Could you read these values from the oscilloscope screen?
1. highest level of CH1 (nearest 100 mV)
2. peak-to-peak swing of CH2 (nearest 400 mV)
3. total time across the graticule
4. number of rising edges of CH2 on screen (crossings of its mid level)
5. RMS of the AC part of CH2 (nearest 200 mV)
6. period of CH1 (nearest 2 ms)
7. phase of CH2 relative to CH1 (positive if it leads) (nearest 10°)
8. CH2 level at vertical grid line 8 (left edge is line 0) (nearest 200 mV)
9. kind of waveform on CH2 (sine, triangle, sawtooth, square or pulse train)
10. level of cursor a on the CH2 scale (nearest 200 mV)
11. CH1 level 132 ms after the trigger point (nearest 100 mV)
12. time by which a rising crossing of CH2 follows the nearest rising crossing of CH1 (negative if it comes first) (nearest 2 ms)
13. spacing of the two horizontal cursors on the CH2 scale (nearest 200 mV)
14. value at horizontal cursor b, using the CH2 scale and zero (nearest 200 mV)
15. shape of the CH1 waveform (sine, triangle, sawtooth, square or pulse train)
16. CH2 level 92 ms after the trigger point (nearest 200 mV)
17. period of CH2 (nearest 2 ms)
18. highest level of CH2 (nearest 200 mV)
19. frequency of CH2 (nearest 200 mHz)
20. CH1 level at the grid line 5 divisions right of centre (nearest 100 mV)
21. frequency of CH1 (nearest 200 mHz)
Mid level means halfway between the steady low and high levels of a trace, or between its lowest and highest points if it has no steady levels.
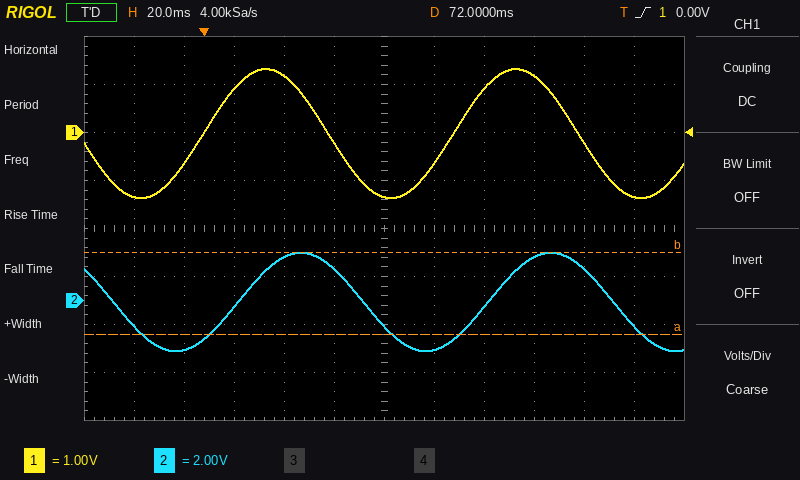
1.3 V
4.0 V
240 ms
2
1.4 V
100 ms
-50°
-200 mV
sine
-1.4 V
1.2 V
+14 ms
3.4 V
2.0 V
sine
-2.0 V
100 ms
2.0 V
10.0 Hz
-1.3 V
10.0 Hz
